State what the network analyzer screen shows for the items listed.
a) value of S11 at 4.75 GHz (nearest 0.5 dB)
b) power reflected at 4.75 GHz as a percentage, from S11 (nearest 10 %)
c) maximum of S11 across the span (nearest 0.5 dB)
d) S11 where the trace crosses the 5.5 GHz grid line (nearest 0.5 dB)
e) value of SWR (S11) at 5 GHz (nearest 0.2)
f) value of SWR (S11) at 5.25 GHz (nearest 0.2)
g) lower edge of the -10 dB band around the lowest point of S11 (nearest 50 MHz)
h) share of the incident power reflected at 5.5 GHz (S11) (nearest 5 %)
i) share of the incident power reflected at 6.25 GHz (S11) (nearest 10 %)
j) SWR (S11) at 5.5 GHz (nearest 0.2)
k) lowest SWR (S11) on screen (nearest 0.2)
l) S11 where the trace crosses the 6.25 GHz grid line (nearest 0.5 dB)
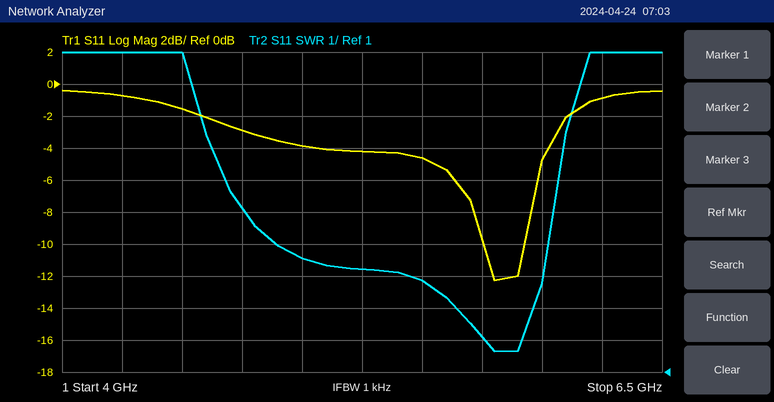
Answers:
-3.0 dB
50 %
-0.5 dB
-4.5 dB
4.6
4.2
5.75 GHz
35 %
80 %
3.8
1.6
-1.0 dB
